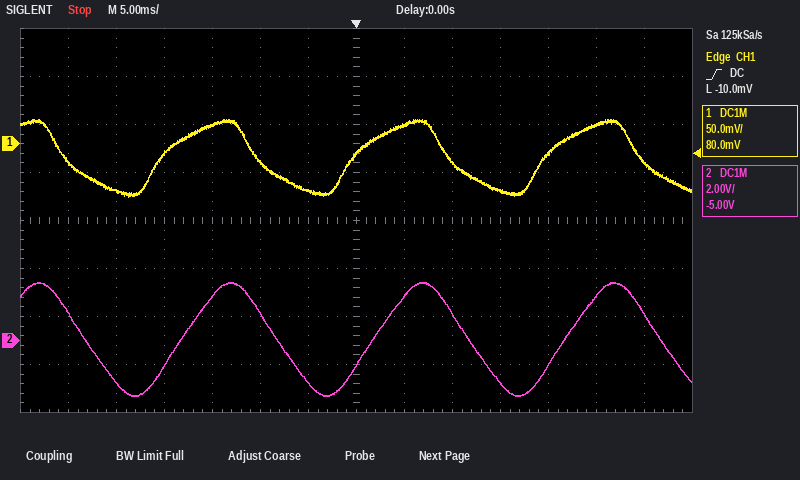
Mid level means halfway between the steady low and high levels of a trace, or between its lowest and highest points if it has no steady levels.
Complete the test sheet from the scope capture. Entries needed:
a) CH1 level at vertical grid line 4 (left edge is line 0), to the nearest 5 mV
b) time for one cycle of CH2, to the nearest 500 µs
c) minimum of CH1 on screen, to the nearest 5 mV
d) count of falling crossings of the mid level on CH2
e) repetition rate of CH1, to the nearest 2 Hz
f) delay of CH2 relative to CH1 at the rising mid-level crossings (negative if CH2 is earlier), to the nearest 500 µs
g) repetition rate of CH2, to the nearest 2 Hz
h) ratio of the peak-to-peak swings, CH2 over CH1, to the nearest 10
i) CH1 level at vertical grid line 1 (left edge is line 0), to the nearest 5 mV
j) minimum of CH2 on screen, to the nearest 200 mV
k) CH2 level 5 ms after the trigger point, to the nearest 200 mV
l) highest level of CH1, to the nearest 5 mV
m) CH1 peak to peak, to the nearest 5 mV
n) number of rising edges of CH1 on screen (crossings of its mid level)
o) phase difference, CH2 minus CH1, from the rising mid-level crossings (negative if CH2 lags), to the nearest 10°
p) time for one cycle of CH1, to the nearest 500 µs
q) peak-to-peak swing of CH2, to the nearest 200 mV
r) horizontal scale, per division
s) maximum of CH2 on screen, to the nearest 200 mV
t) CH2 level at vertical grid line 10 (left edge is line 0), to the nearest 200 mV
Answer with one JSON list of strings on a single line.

["20 mV", "20.0 ms", "-55 mV", "4", "50 Hz", "+2.0 ms", "50 Hz", "60", "-20 mV", "-2.4 V", "1.8 V", "25 mV", "80 mV", "3", "-40°", "20.0 ms", "4.8 V", "5 ms", "2.4 V", "-1.8 V"]
